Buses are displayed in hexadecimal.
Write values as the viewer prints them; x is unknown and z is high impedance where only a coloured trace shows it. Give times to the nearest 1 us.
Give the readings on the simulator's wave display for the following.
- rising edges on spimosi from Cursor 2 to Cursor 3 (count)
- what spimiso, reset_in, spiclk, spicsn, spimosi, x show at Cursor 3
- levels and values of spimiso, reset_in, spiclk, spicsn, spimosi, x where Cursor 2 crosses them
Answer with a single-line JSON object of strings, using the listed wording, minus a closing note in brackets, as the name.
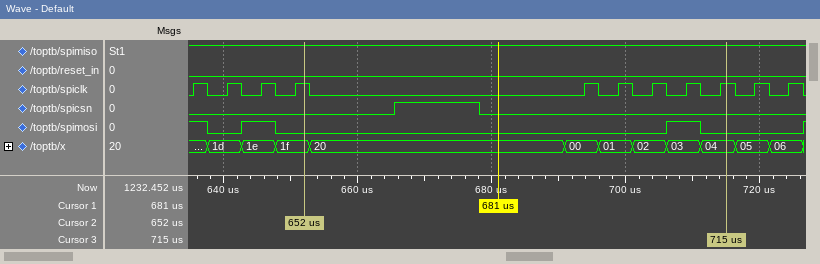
{"rising edges on spimosi from Cursor 2 to Cursor 3": "1", "what spimiso, reset_in, spiclk, spicsn, spimosi, x show at Cursor 3": "spimiso=1, reset_in=0, spiclk=1, spicsn=0, spimosi=0, x=04", "levels and values of spimiso, reset_in, spiclk, spicsn, spimosi, x where Cursor 2 crosses them": "spimiso=1, reset_in=0, spiclk=1, spicsn=0, spimosi=0, x=1f"}
